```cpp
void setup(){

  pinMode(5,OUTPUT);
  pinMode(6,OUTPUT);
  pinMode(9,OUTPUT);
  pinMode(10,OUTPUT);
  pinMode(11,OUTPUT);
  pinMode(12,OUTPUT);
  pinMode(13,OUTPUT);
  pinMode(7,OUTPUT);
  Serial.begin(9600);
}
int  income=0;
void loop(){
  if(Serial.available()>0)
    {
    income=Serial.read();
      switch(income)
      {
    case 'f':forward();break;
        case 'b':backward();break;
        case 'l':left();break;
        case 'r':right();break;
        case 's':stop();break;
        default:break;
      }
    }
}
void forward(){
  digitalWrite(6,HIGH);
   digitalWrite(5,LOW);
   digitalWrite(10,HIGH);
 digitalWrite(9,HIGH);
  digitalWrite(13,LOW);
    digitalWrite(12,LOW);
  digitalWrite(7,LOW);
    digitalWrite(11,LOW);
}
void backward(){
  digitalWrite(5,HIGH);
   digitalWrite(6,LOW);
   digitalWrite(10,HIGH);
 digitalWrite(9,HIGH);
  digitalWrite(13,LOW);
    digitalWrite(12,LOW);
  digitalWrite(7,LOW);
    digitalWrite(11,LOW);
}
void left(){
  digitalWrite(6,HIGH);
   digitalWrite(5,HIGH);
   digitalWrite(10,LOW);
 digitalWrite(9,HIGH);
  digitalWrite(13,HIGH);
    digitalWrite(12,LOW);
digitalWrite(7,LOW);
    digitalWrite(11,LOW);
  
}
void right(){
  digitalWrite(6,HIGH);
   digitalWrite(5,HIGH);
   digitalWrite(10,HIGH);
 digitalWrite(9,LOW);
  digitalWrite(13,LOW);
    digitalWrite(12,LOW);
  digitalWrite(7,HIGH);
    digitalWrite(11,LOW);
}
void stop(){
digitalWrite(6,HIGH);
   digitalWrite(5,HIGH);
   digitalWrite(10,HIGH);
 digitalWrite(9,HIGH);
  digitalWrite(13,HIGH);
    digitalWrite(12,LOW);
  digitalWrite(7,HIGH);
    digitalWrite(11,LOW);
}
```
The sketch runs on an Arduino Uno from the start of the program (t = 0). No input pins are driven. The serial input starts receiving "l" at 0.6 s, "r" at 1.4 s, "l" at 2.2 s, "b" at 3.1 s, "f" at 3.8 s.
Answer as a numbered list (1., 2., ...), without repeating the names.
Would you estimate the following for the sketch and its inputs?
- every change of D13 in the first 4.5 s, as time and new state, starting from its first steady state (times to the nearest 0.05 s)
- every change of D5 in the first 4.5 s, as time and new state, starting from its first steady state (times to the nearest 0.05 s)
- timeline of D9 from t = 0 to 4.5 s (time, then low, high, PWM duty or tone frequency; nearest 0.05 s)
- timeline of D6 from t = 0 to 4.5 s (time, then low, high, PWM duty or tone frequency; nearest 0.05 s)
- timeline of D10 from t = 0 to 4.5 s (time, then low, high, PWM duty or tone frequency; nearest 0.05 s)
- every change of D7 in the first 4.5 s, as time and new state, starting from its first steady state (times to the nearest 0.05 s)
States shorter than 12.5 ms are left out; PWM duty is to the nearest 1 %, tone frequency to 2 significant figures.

1. 0 s low; 0.6 s high; 1.4 s low; 2.2 s high; 3.1 s low
2. 0 s low; 0.6 s high; 3.8 s low
3. 0 s low; 0.6 s high; 1.4 s low; 2.2 s high
4. 0 s low; 0.6 s high; 3.1 s low; 3.8 s high
5. 0 s low; 1.4 s high; 2.2 s low; 3.1 s high
6. 0 s low; 1.4 s high; 2.2 s low
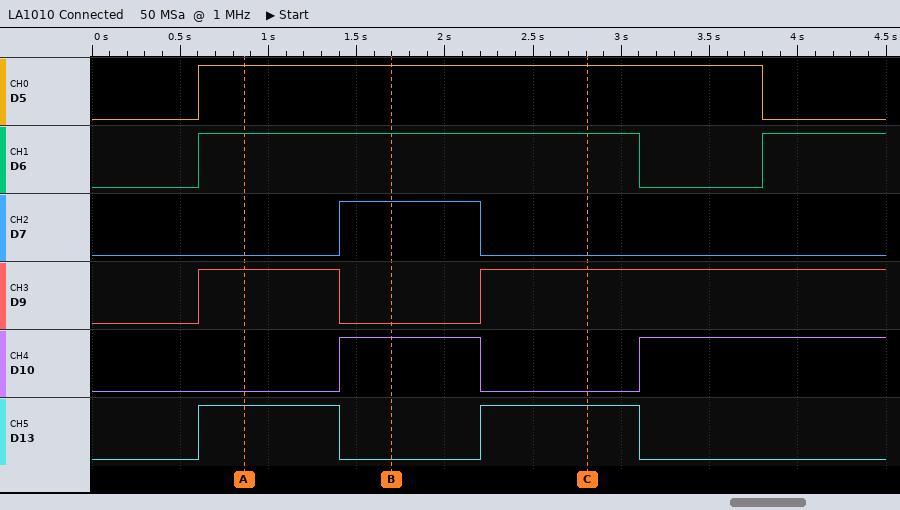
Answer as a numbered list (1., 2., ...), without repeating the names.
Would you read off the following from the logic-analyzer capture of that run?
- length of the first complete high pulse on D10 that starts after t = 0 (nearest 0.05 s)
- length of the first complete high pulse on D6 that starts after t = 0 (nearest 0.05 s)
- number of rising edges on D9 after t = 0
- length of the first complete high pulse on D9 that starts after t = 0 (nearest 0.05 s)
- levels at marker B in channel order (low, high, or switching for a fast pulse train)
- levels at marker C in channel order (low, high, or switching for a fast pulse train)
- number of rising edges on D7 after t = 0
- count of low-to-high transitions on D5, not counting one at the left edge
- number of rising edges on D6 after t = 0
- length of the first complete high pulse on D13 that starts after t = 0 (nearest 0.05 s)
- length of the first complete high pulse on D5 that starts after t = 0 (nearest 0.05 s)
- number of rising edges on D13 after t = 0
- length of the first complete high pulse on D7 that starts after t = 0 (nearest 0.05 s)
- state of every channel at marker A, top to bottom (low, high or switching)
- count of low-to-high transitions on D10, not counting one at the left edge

1. 0.80 s
2. 2.50 s
3. 2
4. 0.80 s
5. D5 high, D6 high, D7 high, D9 low, D10 high, D13 low
6. D5 high, D6 high, D7 low, D9 high, D10 low, D13 high
7. 1
8. 1
9. 2
10. 0.80 s
11. 3.20 s
12. 2
13. 0.80 s
14. D5 high, D6 high, D7 low, D9 high, D10 low, D13 high
15. 2
